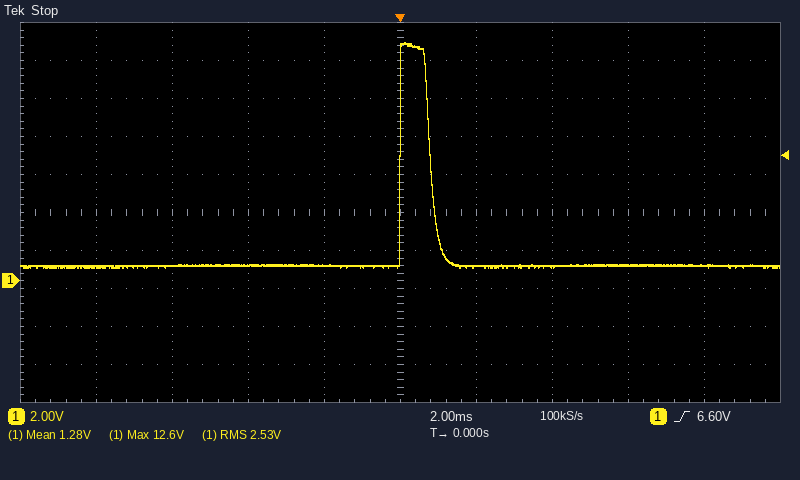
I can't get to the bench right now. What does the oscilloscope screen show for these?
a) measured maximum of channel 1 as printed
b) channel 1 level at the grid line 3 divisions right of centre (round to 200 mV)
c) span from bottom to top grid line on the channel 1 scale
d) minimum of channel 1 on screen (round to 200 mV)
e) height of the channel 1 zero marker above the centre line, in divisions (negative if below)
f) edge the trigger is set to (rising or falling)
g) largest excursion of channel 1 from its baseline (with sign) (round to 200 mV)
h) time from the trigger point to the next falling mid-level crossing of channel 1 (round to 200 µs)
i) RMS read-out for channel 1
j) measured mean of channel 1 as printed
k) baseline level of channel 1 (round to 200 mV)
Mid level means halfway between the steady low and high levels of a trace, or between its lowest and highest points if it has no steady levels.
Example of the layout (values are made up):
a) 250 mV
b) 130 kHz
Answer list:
a) 12.6 V
b) 800 mV
c) 20 V
d) 800 mV
e) -1.8 div
f) rising
g) +11.8 V
h) 800 µs
i) 2.53 V
j) 1.28 V
k) 800 mV
